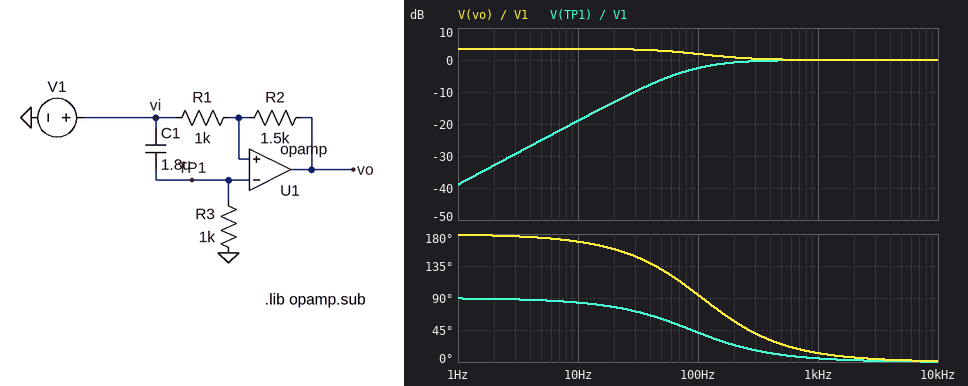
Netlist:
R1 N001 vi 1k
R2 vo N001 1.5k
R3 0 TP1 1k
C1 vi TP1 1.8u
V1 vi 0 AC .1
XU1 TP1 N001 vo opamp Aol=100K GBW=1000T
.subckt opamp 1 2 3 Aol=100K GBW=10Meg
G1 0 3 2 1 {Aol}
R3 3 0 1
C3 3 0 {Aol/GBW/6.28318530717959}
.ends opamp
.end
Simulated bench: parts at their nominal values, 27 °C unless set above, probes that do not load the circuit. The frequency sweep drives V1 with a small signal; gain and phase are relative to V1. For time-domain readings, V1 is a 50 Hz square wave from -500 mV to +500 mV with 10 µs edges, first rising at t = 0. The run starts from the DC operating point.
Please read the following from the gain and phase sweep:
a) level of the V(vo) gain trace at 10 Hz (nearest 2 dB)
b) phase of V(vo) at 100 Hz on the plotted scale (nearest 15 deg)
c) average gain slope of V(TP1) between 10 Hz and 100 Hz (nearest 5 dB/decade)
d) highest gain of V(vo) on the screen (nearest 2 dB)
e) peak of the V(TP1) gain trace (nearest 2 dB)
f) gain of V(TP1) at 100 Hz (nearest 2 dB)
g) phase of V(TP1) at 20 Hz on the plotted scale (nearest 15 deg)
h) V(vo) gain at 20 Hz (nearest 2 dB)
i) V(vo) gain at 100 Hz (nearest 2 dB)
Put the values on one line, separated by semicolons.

4 dB; 90 deg; 15 dB/decade; 4 dB; 0 dB; -2 dB; 75 deg; 4 dB; 2 dB
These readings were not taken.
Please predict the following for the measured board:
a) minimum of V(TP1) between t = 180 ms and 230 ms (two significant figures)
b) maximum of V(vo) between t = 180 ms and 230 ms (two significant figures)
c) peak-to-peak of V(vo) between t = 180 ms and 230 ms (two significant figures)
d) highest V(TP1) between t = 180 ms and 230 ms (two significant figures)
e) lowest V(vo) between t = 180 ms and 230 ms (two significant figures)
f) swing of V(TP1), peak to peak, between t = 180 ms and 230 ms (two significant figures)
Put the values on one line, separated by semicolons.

-990 mV; 1.7 V; 3.5 V; 990 mV; -1.7 V; 2.0 V
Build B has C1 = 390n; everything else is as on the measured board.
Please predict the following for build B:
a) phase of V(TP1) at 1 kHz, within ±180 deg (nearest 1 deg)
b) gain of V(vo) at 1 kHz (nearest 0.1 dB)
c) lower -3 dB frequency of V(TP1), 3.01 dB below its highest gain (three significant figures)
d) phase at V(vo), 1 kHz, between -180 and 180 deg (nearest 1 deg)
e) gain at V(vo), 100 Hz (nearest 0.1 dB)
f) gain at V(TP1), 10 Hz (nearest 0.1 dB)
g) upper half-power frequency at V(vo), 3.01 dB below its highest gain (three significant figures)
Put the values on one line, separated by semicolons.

22 deg; 0.7 dB; 408 Hz; 54 deg; 3.4 dB; -32.2 dB; 1.22 kHz
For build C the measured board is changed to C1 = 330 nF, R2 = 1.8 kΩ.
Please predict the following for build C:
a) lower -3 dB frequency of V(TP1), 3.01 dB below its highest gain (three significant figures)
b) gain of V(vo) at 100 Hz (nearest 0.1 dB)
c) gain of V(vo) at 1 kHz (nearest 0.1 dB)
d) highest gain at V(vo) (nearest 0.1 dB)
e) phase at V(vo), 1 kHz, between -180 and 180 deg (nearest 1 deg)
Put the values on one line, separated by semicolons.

482 Hz; 5.0 dB; 1.5 dB; 5.1 dB; 67 deg
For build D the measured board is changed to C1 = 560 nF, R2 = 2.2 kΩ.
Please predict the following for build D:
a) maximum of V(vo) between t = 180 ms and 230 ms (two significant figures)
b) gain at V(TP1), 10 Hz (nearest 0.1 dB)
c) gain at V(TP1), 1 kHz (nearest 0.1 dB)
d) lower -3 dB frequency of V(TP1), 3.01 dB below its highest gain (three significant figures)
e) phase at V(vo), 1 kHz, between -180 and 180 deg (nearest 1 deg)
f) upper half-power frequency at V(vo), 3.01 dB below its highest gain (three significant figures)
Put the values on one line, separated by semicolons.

2.1 V; -29.1 dB; -0.3 dB; 284 Hz; 48 deg; 371 Hz
